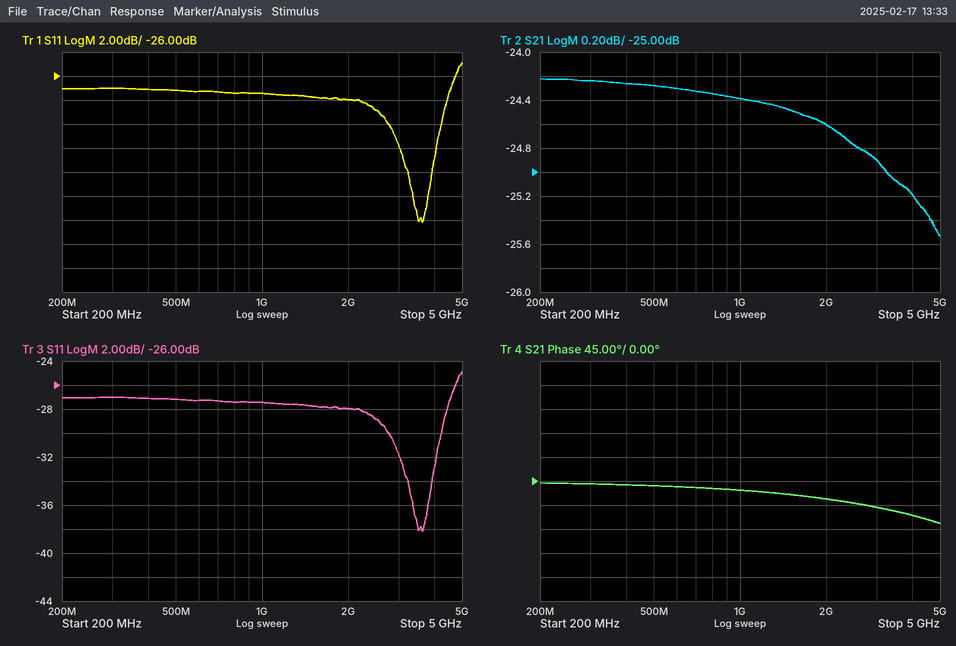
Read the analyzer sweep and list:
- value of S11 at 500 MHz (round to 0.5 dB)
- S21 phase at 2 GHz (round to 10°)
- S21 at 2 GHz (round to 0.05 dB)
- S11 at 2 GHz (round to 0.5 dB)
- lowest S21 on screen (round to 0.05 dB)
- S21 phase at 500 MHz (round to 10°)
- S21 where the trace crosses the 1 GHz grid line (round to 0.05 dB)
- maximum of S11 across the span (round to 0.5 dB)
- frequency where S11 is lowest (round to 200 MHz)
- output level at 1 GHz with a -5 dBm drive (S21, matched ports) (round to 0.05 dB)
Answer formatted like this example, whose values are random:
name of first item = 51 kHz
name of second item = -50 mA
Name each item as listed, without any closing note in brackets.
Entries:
value of S11 at 500 MHz = -27.0 dB
S21 phase at 2 GHz = -30°
S21 at 2 GHz = -24.60 dB
S11 at 2 GHz = -28.0 dB
lowest S21 on screen = -25.55 dB
S21 phase at 500 MHz = -10°
S21 where the trace crosses the 1 GHz grid line = -24.40 dB
maximum of S11 across the span = -25.0 dB
frequency where S11 is lowest = 3.6 GHz
output level at 1 GHz with a -5 dBm drive (S21, matched ports) = -29.40 dBm
